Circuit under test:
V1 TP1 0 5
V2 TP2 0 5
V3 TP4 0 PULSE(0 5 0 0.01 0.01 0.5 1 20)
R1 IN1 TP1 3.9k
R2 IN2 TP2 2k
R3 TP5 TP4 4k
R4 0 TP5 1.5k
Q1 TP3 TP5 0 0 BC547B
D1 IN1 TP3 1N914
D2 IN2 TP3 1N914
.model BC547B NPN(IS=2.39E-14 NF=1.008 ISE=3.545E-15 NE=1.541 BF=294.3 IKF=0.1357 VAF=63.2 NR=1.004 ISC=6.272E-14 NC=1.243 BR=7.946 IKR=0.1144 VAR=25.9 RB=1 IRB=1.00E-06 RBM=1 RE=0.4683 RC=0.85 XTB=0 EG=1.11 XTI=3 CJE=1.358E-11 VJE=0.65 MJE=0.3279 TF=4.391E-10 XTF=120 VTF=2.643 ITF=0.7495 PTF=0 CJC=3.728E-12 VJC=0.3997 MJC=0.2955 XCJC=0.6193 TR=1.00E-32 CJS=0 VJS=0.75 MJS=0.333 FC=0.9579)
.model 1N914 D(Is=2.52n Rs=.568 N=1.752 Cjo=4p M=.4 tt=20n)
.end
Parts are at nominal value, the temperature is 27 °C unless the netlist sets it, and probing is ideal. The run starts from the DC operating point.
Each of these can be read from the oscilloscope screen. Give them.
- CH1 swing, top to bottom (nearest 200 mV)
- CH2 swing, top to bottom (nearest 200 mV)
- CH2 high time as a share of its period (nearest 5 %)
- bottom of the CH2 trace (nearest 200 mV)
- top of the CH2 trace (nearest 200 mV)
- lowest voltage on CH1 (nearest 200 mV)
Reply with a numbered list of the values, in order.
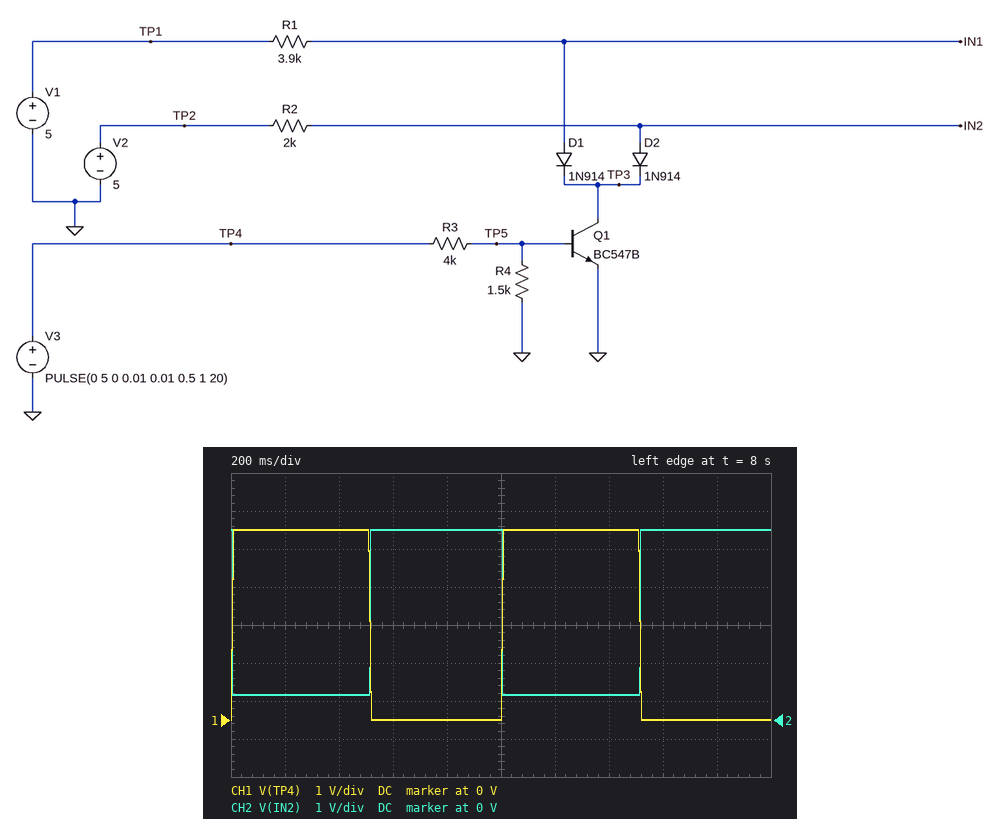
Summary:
1. 5.0 V
2. 4.4 V
3. 50 %
4. 600 mV
5. 5.0 V
6. 0 V
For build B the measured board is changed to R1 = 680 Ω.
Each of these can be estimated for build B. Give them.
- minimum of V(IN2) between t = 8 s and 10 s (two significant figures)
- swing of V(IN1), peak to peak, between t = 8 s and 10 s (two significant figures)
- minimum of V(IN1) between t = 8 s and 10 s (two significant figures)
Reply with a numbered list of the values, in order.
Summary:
1. 670 mV
2. 4.3 V
3. 720 mV
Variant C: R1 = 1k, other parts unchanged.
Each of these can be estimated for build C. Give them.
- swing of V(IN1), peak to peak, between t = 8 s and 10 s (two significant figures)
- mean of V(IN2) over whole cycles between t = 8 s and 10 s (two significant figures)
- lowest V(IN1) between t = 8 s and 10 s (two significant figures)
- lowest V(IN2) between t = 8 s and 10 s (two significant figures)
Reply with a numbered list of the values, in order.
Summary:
1. 4.3 V
2. 2.8 V
3. 690 mV
4. 660 mV
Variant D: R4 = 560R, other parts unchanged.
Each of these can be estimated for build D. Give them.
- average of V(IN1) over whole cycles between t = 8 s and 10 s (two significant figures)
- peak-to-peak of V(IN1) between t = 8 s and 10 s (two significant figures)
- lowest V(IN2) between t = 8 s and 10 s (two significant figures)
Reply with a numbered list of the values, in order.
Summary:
1. 4.7 V
2. 550 mV
3. 4.5 V
